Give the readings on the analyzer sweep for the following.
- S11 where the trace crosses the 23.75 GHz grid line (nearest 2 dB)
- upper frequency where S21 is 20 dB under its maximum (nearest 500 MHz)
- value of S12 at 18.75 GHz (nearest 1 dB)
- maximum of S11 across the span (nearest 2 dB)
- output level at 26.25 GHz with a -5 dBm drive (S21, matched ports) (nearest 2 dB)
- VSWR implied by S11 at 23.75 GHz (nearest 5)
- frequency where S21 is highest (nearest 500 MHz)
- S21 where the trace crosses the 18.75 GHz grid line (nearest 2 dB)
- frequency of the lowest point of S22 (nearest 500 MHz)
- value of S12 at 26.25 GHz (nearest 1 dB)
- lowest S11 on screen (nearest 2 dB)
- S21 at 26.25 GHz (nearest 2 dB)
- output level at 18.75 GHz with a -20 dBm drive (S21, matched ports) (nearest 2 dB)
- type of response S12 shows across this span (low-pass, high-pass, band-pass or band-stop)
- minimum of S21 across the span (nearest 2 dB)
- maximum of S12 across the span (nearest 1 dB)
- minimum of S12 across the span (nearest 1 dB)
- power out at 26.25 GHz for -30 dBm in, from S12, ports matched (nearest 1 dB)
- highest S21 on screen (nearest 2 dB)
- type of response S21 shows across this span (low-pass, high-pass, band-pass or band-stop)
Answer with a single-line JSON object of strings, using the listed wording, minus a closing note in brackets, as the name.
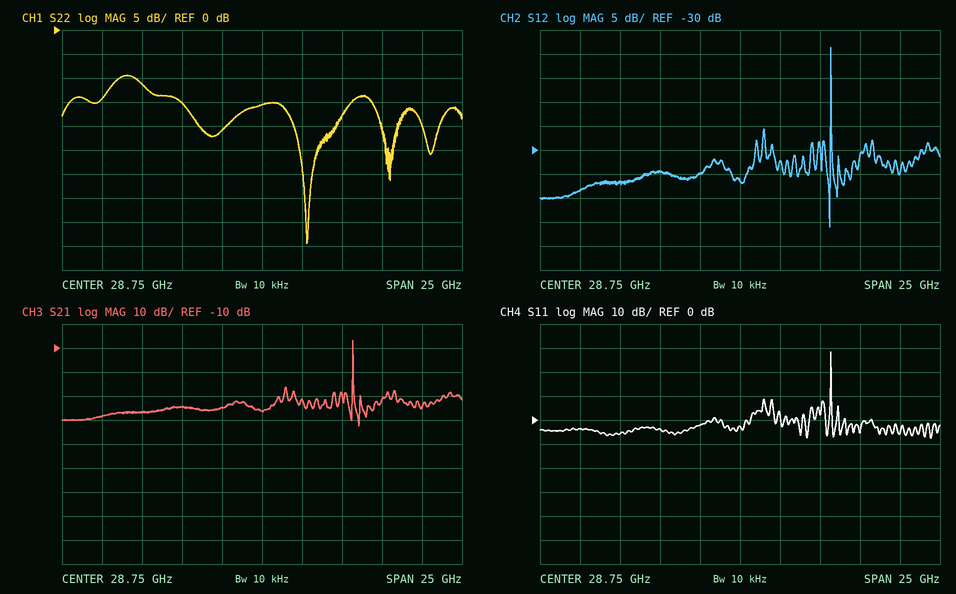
{"S11 where the trace crosses the 23.75 GHz grid line": "-4 dB", "upper frequency where S21 is 20 dB under its maximum": "34.5 GHz", "value of S12 at 18.75 GHz": "-38 dB", "maximum of S11 across the span": "28 dB", "output level at 26.25 GHz with a -5 dBm drive (S21, matched ports)": "-40 dBm", "VSWR implied by S11 at 23.75 GHz": "5", "frequency where S21 is highest": "34.5 GHz", "S21 where the trace crosses the 18.75 GHz grid line": "-38 dB", "frequency of the lowest point of S22": "31.5 GHz", "value of S12 at 26.25 GHz": "-35 dB", "lowest S11 on screen": "-8 dB", "S21 at 26.25 GHz": "-34 dB", "output level at 18.75 GHz with a -20 dBm drive (S21, matched ports)": "-58 dBm", "type of response S12 shows across this span": "band-pass", "minimum of S21 across the span": "-42 dB", "maximum of S12 across the span": "-9 dB", "minimum of S12 across the span": "-46 dB", "power out at 26.25 GHz for -30 dBm in, from S12, ports matched": "-65 dBm", "highest S21 on screen": "-6 dB", "type of response S21 shows across this span": "band-pass"}
